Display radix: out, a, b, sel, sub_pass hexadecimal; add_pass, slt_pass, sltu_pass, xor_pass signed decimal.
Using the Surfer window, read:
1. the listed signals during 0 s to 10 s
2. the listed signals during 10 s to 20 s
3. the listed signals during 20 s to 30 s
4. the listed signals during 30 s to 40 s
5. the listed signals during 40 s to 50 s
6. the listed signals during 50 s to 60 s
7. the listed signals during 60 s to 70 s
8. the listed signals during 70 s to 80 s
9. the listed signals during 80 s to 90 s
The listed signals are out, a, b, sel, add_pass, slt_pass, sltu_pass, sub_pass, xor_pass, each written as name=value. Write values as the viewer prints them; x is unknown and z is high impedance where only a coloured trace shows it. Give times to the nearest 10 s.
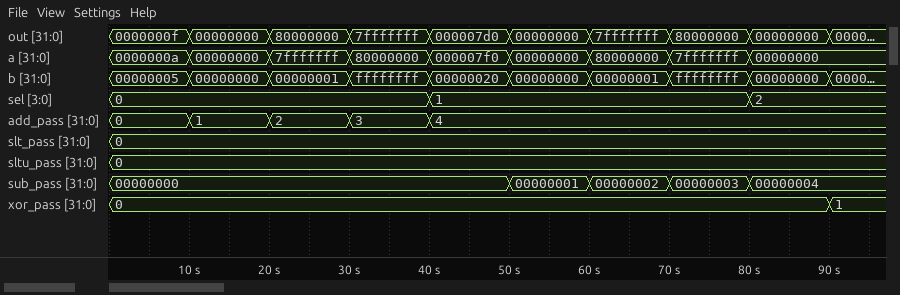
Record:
out=0000000f, a=0000000a, b=00000005, sel=0, add_pass=0, slt_pass=0, sltu_pass=0, sub_pass=00000000, xor_pass=0
out=00000000, a=00000000, b=00000000, sel=0, add_pass=1, slt_pass=0, sltu_pass=0, sub_pass=00000000, xor_pass=0
out=80000000, a=7fffffff, b=00000001, sel=0, add_pass=2, slt_pass=0, sltu_pass=0, sub_pass=00000000, xor_pass=0
out=7fffffff, a=80000000, b=ffffffff, sel=0, add_pass=3, slt_pass=0, sltu_pass=0, sub_pass=00000000, xor_pass=0
out=000007d0, a=000007f0, b=00000020, sel=1, add_pass=4, slt_pass=0, sltu_pass=0, sub_pass=00000000, xor_pass=0
out=00000000, a=00000000, b=00000000, sel=1, add_pass=4, slt_pass=0, sltu_pass=0, sub_pass=00000001, xor_pass=0
out=7fffffff, a=80000000, b=00000001, sel=1, add_pass=4, slt_pass=0, sltu_pass=0, sub_pass=00000002, xor_pass=0
out=80000000, a=7fffffff, b=ffffffff, sel=1, add_pass=4, slt_pass=0, sltu_pass=0, sub_pass=00000003, xor_pass=0
out=00000000, a=00000000, b=00000000, sel=2, add_pass=4, slt_pass=0, sltu_pass=0, sub_pass=00000004, xor_pass=0
